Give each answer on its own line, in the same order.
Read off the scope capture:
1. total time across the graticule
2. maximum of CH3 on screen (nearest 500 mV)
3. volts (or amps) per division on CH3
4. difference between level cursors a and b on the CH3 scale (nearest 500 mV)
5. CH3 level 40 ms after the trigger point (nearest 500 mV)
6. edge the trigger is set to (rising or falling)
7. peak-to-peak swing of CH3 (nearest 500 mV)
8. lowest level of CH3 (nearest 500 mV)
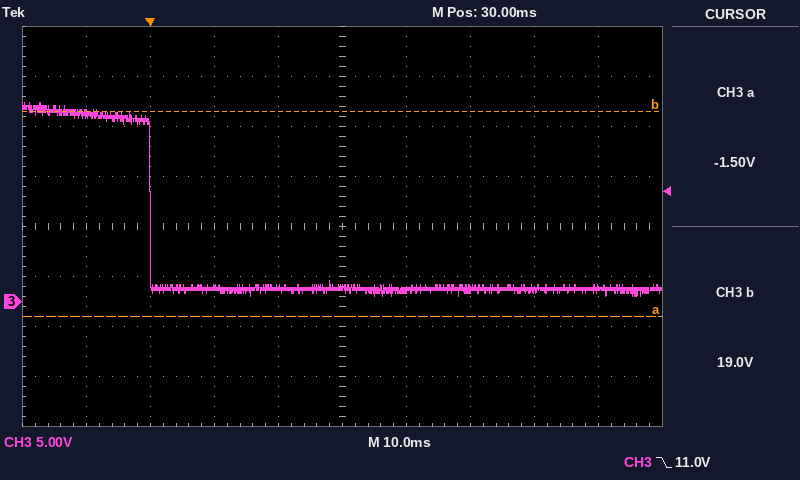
100 ms
20.0 V
5 V
20.5 V
1.0 V
falling
19.5 V
500 mV
